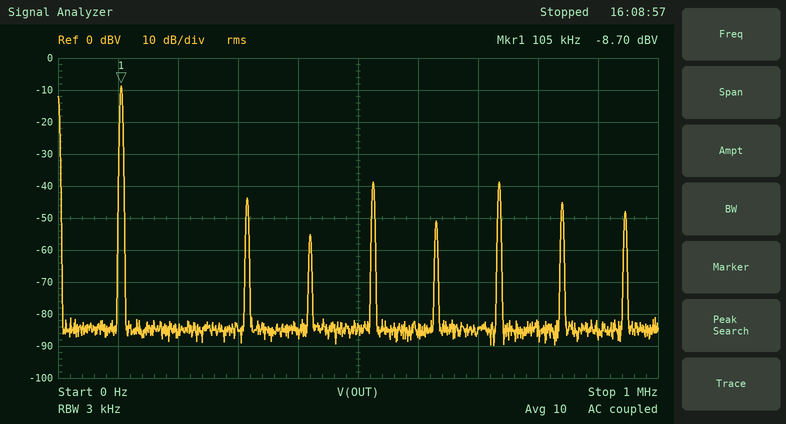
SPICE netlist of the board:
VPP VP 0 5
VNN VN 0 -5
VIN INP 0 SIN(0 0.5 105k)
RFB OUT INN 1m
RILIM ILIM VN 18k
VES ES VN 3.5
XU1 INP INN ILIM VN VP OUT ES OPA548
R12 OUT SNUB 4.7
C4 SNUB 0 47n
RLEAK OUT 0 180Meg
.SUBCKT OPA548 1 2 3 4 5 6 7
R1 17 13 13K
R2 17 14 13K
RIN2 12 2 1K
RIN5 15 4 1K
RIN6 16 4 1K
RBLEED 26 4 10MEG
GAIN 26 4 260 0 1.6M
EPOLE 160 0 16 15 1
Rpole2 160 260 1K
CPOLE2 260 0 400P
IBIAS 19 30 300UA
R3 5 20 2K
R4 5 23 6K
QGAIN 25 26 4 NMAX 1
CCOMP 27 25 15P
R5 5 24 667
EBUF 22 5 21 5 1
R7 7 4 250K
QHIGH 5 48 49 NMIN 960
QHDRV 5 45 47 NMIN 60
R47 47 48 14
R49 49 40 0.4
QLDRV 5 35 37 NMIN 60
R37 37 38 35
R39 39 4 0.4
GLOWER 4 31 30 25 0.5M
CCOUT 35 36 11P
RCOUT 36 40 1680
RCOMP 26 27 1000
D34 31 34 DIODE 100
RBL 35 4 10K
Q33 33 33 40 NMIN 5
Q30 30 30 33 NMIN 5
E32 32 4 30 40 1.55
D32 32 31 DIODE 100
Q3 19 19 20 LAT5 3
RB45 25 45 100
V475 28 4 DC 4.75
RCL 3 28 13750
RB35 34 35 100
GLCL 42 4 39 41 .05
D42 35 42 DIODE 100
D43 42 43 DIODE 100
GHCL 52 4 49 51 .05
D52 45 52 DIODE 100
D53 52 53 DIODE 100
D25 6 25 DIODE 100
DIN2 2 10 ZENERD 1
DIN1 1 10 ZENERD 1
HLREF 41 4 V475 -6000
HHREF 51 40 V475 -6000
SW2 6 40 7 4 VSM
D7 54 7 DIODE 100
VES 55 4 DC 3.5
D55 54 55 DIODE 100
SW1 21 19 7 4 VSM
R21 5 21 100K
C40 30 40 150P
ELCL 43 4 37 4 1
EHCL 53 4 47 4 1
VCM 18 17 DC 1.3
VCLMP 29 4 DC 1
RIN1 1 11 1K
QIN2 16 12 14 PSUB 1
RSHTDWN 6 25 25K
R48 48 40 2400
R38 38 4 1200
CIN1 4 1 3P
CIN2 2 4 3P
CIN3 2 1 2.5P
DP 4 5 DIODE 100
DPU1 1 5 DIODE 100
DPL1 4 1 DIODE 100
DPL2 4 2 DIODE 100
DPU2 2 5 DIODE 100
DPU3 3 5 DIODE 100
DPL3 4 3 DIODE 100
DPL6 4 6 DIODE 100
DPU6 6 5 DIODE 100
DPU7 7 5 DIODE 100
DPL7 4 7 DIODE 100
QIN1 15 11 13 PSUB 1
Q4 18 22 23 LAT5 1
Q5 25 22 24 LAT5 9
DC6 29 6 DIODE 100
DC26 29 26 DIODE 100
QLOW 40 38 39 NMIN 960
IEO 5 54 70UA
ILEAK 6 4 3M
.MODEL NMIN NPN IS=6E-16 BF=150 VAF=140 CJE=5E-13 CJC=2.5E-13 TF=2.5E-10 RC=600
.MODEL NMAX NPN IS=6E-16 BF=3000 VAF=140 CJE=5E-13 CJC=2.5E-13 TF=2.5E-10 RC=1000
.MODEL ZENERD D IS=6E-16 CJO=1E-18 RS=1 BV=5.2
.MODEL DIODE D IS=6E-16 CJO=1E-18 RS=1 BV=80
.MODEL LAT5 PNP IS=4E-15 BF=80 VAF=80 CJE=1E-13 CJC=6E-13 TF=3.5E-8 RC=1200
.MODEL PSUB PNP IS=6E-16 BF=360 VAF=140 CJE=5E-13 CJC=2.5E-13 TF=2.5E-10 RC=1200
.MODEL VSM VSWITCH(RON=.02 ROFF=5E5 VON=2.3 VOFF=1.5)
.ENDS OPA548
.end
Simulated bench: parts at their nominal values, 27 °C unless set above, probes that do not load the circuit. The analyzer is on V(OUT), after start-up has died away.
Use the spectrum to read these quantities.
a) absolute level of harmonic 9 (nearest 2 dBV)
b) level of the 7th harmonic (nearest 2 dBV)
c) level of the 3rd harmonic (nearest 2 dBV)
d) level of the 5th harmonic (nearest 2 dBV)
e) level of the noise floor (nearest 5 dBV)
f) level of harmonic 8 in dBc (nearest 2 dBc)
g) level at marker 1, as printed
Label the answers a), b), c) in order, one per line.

a) -48 dBV
b) -38 dBV
c) -44 dBV
d) -38 dBV
e) -85 dBV
f) -36 dBc
g) -8.70 dBV
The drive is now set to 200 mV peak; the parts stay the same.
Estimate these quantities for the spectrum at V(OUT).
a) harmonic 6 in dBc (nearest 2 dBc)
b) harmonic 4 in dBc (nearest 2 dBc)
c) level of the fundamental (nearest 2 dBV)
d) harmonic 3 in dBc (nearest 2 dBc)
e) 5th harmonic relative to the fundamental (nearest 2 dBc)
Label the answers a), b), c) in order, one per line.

a) -28 dBc
b) -28 dBc
c) -16 dBV
d) -44 dBc
e) -22 dBc
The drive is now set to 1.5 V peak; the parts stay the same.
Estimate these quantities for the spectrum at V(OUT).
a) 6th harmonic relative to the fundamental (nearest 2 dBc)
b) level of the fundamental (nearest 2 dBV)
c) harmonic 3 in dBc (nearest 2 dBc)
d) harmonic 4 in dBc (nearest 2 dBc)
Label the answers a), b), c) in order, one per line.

a) -46 dBc
b) 0 dBV
c) -42 dBc
d) -56 dBc
